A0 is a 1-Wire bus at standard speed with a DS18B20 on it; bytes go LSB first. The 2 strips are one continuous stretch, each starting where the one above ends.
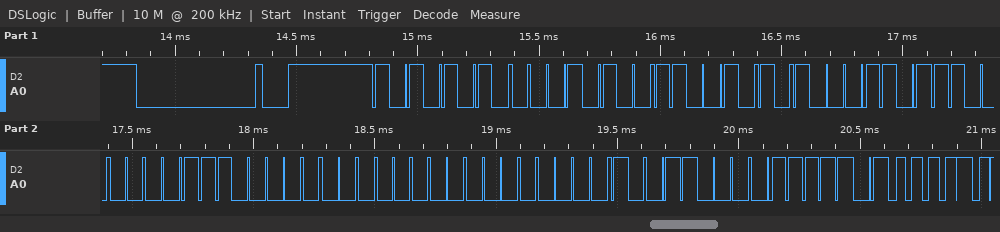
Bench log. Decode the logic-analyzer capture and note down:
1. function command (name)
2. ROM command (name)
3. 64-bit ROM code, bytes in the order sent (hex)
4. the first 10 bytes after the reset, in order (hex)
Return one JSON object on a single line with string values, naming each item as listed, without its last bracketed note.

{"function command": "Read Scratchpad", "ROM command": "Match ROM", "64-bit ROM code, bytes in the order sent": "28 53 B1 03 07 00 00 19", "the first 10 bytes after the reset, in order": "55 28 53 B1 03 07 00 00 19 BE"}
